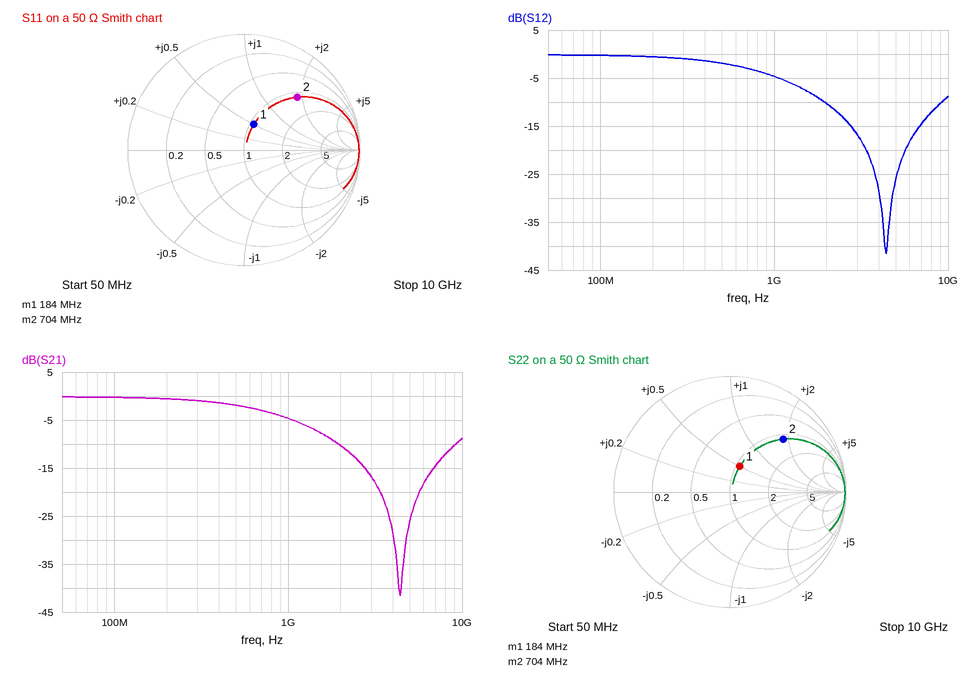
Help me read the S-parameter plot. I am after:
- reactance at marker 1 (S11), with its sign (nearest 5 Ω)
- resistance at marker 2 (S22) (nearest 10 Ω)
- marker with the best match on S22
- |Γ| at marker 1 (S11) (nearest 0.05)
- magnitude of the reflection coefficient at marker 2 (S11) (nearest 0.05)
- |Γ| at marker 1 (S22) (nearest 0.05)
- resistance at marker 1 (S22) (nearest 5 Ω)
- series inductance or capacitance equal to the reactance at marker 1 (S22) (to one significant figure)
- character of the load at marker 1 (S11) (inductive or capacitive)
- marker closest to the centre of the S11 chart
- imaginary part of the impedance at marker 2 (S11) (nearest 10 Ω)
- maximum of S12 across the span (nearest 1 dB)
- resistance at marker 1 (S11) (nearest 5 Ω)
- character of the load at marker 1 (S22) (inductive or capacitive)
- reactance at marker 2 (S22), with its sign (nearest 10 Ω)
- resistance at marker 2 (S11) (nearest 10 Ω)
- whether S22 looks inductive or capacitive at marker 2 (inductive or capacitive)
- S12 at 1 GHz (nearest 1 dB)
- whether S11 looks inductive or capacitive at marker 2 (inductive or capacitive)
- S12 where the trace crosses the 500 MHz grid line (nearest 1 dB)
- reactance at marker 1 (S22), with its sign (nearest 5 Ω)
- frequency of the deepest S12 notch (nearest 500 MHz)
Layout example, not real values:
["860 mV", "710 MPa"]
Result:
["+25 Ω", "60 Ω", "marker 1", "0.25", "0.65", "0.25", "55 Ω", "20 nH", "inductive", "marker 1", "+90 Ω", "0 dB", "55 Ω", "inductive", "+90 Ω", "60 Ω", "inductive", "-5 dB", "inductive", "-2 dB", "+25 Ω", "4.5 GHz"]
